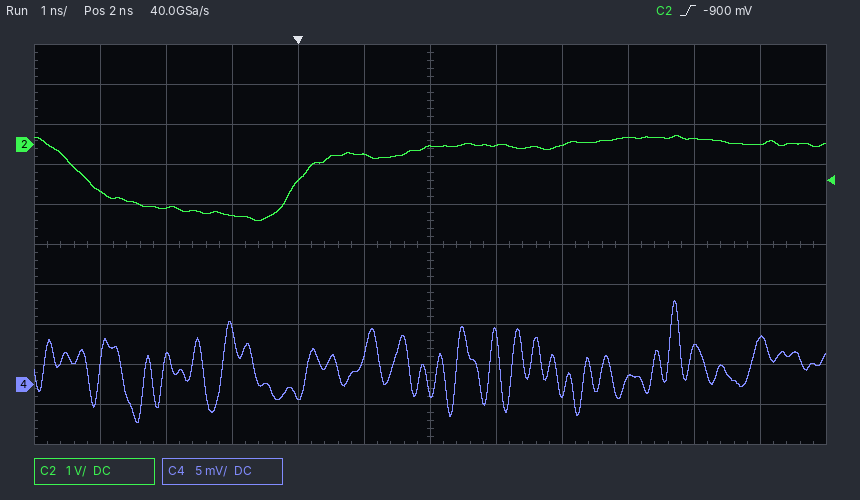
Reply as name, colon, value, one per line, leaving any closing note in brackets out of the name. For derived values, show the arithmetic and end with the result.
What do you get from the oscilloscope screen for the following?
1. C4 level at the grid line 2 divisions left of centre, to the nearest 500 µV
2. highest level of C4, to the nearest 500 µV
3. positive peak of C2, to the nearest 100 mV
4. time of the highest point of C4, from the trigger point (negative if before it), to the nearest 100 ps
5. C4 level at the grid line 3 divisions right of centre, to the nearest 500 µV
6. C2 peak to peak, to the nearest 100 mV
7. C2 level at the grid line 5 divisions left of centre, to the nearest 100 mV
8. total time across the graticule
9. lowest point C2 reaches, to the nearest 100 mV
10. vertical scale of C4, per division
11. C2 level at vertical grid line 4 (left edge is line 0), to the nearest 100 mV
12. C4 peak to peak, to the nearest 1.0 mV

C4 level at the grid line 2 divisions left of centre, to the nearest 500 µV: -1.5 mV
highest level of C4, to the nearest 500 µV: 10.5 mV
positive peak of C2, to the nearest 100 mV: 200 mV
time of the highest point of C4, from the trigger point (negative if before it), to the nearest 100 ps: +5.7 ns
C4 level at the grid line 3 divisions right of centre, to the nearest 500 µV: 1.0 mV
C2 peak to peak, to the nearest 100 mV: 200 mV − (-1.9 V) = 2.1 V
C2 level at the grid line 5 divisions left of centre, to the nearest 100 mV: -1.2 V
total time across the graticule: 12 ns
lowest point C2 reaches, to the nearest 100 mV: -1.9 V
vertical scale of C4, per division: 5 mV
C2 level at vertical grid line 4 (left edge is line 0), to the nearest 100 mV: -900 mV
C4 peak to peak, to the nearest 1.0 mV: 15.0 mV
